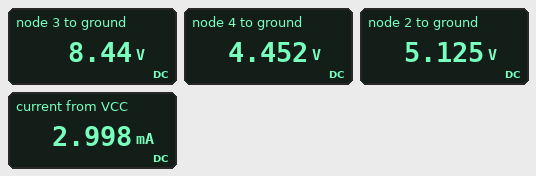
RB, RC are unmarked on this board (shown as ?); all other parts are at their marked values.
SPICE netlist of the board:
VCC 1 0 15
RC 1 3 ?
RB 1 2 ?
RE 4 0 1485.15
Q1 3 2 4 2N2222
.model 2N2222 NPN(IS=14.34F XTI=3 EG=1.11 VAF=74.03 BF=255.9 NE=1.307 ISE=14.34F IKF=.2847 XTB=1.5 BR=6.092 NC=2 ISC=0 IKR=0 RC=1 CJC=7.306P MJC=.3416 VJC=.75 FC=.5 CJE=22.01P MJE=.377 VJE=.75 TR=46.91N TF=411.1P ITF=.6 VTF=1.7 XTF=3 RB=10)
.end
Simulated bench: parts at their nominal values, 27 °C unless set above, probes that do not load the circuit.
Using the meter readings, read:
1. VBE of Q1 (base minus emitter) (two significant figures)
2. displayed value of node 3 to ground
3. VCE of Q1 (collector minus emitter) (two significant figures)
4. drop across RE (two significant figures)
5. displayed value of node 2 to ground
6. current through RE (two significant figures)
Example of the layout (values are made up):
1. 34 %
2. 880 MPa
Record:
1. 670 mV
2. 8.44 V
3. 4.0 V
4. 4.5 V
5. 5.125 V
6. 3.0 mA
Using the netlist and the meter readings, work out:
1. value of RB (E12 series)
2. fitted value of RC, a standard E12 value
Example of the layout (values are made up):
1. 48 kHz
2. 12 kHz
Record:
1. 560 kΩ
2. 2.2 kΩ
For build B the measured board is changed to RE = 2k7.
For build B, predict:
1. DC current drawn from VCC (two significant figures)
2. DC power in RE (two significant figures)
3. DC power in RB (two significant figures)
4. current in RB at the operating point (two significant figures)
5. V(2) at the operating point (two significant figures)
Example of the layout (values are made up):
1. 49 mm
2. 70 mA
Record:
1. 2.4 mA
2. 15 mW
3. 110 µW
4. 14 µA
5. 7.0 V
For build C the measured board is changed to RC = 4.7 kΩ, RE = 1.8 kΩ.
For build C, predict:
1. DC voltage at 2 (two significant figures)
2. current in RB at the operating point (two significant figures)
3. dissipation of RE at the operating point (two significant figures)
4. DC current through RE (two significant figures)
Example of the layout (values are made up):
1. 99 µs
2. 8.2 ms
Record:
1. 4.8 V
2. 18 µA
3. 9.5 mW
4. 2.3 mA
